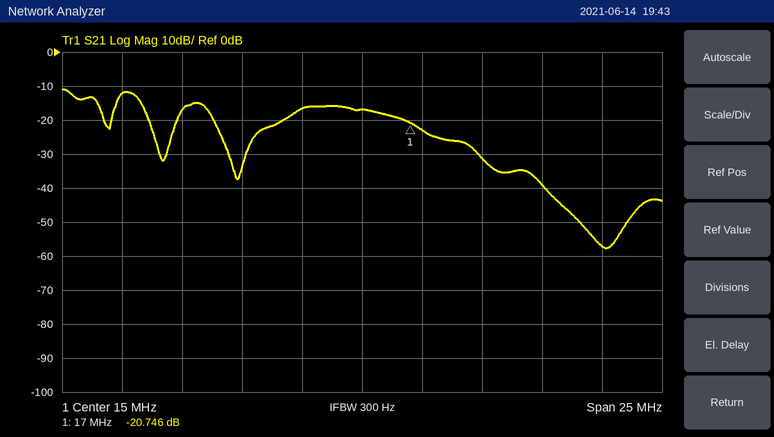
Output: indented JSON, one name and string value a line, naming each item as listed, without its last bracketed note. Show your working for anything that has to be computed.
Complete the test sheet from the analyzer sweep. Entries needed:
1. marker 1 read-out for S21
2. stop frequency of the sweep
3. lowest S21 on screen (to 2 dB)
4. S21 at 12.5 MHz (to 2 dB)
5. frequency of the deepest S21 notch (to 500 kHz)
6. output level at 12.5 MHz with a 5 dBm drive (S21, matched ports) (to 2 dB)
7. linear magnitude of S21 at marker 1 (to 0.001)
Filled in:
{
  "marker 1 read-out for S21": "-20.746 dB",
  "stop frequency of the sweep": "27.5 MHz",
  "lowest S21 on screen": "-58 dB",
  "S21 at 12.5 MHz": "-16 dB",
  "frequency of the deepest S21 notch": "25.0 MHz",
  "output level at 12.5 MHz with a 5 dBm drive (S21, matched ports)": "5 dBm + (-16 dB) = -12 dBm",
  "linear magnitude of S21 at marker 1": "10^(-20.746/20) ≈ 0.092"
}
